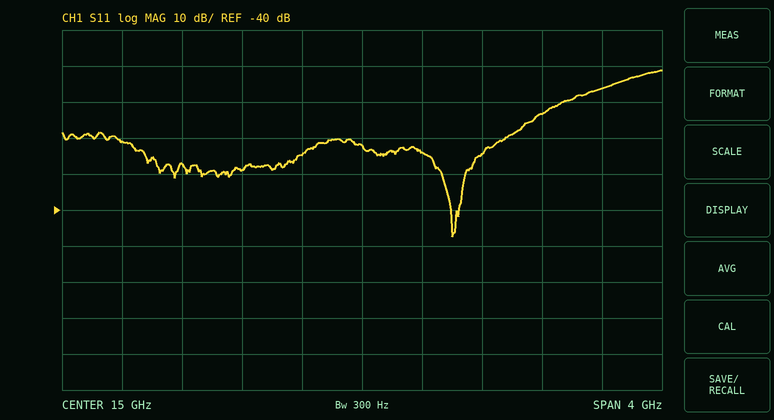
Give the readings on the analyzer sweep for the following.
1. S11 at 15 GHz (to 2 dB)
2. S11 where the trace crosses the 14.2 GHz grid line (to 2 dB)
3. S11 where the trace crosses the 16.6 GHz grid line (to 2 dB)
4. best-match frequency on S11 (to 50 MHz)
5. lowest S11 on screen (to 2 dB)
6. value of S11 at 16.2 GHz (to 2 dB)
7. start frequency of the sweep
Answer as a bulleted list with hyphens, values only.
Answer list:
- -22 dB
- -28 dB
- -6 dB
- 15.60 GHz
- -48 dB
- -14 dB
- 13 GHz
